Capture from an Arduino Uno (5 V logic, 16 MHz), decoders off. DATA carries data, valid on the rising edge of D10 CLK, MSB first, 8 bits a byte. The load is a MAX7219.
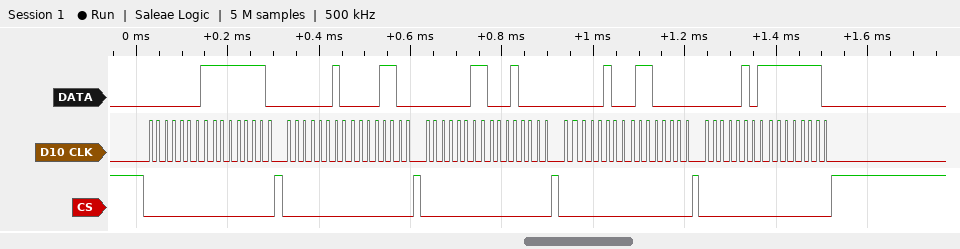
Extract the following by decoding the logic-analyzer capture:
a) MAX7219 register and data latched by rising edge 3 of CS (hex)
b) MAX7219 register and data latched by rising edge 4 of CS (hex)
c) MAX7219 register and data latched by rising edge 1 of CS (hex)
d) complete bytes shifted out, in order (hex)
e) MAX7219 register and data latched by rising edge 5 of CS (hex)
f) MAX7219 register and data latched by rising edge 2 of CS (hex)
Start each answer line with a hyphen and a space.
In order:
- register 0x3, data 0x10
- register 0x4, data 0x60
- register 0x1, data 0xFE
- 01 FE 02 0C 03 10 04 60 05 FE
- register 0x5, data 0xFE
- register 0x2, data 0x0C
